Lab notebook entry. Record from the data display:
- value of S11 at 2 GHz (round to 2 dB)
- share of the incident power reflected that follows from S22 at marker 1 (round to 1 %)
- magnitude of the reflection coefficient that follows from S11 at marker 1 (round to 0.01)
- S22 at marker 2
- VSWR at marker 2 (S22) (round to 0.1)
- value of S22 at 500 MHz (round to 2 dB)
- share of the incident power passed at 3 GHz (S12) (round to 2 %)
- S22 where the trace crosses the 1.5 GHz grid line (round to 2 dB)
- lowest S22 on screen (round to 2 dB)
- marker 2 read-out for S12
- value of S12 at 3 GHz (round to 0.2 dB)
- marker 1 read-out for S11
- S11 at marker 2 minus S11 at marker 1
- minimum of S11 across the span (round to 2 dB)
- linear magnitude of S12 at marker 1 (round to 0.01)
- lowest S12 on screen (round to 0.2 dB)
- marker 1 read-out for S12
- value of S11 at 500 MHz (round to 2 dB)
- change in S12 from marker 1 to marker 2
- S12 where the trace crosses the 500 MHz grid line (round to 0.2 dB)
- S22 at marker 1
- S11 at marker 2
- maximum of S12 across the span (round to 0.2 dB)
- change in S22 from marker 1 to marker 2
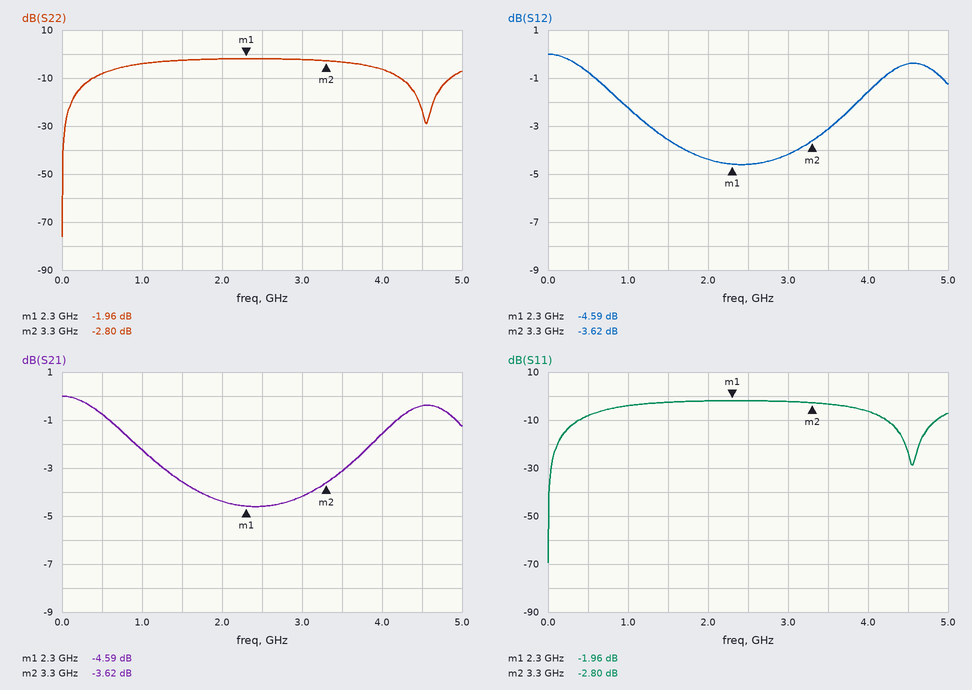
-2 dB
64 %
0.80
-2.80 dB
6.3
-8 dB
38 %
-2 dB
-76 dB
-3.62 dB
-4.2 dB
-1.96 dB
-0.84 dB
-70 dB
0.59
-4.6 dB
-4.59 dB
-8 dB
0.97 dB
-0.8 dB
-1.96 dB
-2.80 dB
0.0 dB
-0.84 dB
